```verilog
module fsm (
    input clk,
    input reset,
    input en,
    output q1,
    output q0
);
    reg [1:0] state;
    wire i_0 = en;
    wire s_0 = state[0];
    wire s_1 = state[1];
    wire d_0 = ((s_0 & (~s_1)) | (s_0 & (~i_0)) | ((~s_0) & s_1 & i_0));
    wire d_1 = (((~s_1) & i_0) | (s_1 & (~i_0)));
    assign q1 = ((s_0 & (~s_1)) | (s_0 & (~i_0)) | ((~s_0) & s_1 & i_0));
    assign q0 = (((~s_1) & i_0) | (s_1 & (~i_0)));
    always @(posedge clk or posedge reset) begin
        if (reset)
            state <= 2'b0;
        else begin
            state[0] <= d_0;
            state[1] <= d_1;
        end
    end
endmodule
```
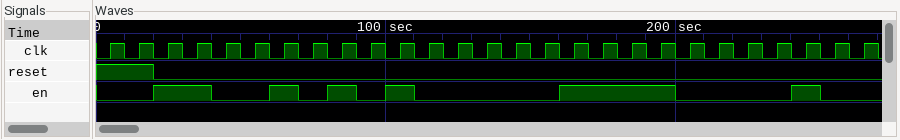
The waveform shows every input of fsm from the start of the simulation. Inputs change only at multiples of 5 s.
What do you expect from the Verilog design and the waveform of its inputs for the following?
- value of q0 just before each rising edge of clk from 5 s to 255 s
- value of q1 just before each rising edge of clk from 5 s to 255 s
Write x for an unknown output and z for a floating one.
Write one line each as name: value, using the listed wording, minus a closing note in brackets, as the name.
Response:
value of q0 just before each rising edge of clk from 5 s to 255 s: 0 0 1 0 0 0 1 1 0 0 1 1 1 1 1 1 0 1 0 1 1 1 1 1 0 0
value of q1 just before each rising edge of clk from 5 s to 255 s: 0 0 0 1 1 1 1 1 0 0 0 0 0 0 0 0 1 1 0 0 0 0 0 0 1 1
